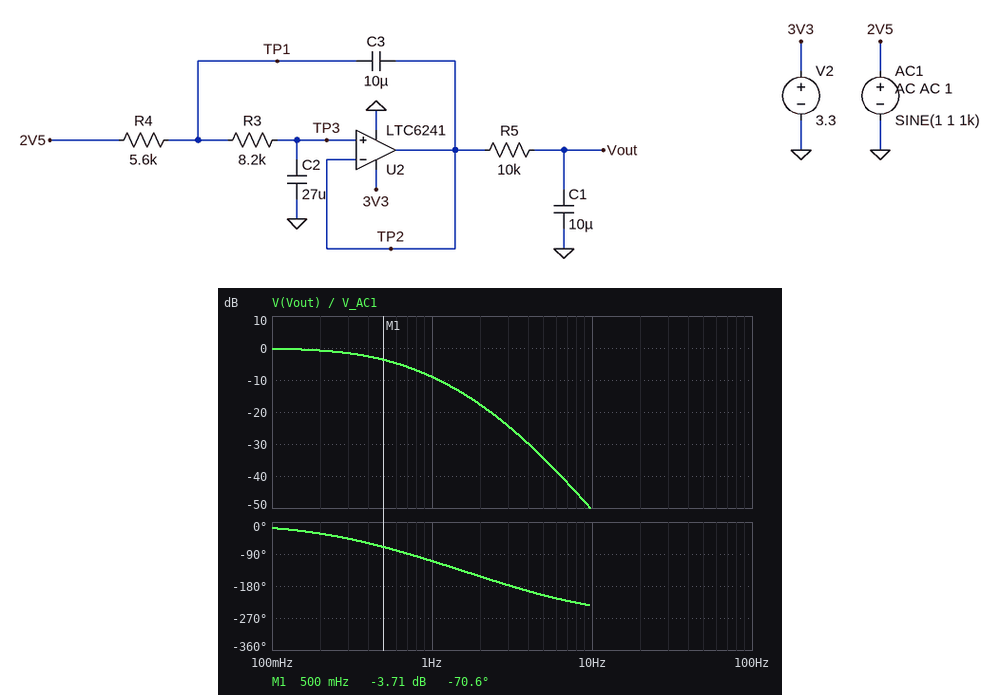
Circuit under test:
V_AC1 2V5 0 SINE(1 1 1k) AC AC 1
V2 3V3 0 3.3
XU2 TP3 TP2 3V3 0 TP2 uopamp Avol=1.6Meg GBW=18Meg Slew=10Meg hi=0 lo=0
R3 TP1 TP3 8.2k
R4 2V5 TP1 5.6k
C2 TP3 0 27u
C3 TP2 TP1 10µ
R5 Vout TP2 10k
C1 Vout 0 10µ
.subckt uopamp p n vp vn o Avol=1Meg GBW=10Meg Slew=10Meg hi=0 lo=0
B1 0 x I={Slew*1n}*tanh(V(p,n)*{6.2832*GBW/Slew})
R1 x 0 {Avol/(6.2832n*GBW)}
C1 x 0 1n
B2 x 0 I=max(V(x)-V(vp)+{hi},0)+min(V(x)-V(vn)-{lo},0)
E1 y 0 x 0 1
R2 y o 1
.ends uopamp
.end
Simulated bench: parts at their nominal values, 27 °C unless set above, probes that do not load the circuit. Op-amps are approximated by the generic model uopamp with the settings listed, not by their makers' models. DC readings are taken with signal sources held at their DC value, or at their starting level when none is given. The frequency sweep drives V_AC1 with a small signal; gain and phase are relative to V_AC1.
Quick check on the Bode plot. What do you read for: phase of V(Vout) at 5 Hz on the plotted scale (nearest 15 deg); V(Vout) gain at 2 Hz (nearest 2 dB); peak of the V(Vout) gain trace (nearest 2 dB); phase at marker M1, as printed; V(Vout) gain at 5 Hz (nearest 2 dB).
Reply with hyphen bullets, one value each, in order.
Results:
- -210 deg
- -18 dB
- 0 dB
- -70.6 deg
- -34 dB
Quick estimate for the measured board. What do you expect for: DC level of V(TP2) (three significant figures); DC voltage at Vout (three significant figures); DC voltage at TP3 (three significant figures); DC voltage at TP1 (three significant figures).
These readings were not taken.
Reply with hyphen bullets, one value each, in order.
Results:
- 1.00 V
- 1.00 V
- 1.00 V
- 1.00 V
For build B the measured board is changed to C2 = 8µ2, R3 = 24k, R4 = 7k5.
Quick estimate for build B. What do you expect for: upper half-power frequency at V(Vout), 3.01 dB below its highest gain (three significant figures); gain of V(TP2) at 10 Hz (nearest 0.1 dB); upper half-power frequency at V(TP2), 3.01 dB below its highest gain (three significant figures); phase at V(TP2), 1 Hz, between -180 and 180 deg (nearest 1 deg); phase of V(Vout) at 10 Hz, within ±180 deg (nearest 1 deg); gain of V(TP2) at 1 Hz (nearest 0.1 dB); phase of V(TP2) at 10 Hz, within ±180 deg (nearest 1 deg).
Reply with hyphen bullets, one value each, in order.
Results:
- 661 mHz
- -35.5 dB
- 773 mHz
- -76 deg
- 115 deg
- -4.5 dB
- -164 deg
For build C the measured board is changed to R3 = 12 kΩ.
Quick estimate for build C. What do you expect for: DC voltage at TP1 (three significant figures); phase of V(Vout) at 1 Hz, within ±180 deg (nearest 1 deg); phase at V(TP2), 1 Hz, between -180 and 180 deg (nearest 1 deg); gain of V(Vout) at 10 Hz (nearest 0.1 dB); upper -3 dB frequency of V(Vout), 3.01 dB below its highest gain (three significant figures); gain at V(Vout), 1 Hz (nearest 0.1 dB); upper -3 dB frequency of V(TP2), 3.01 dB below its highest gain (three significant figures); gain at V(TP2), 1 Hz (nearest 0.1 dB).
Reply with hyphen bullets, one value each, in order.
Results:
- 1.00 V
- -117 deg
- -85 deg
- -53.8 dB
- 347 mHz
- -11.0 dB
- 364 mHz
- -9.5 dB
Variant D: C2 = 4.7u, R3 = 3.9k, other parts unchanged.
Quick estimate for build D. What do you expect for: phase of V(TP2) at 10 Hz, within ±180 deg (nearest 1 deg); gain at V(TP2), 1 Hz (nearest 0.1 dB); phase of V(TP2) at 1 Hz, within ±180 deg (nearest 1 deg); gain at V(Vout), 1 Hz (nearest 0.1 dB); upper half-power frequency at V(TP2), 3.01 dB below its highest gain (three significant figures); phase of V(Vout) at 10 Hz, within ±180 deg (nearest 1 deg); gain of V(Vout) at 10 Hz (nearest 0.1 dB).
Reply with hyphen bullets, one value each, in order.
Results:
- -137 deg
- 0 dB
- -16 deg
- -1.4 dB
- 5.04 Hz
- 142 deg
- -28.4 dB
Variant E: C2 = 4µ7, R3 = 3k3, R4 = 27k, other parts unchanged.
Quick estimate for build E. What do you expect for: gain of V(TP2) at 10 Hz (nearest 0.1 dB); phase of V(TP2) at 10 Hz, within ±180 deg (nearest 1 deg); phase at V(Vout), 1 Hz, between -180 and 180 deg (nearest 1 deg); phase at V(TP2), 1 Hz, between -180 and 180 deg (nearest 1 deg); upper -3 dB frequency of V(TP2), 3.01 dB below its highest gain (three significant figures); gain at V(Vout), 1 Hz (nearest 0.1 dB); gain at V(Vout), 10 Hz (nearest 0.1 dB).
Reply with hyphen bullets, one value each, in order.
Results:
- -25.1 dB
- -150 deg
- -79 deg
- -47 deg
- 1.38 Hz
- -3.2 dB
- -41.1 dB
